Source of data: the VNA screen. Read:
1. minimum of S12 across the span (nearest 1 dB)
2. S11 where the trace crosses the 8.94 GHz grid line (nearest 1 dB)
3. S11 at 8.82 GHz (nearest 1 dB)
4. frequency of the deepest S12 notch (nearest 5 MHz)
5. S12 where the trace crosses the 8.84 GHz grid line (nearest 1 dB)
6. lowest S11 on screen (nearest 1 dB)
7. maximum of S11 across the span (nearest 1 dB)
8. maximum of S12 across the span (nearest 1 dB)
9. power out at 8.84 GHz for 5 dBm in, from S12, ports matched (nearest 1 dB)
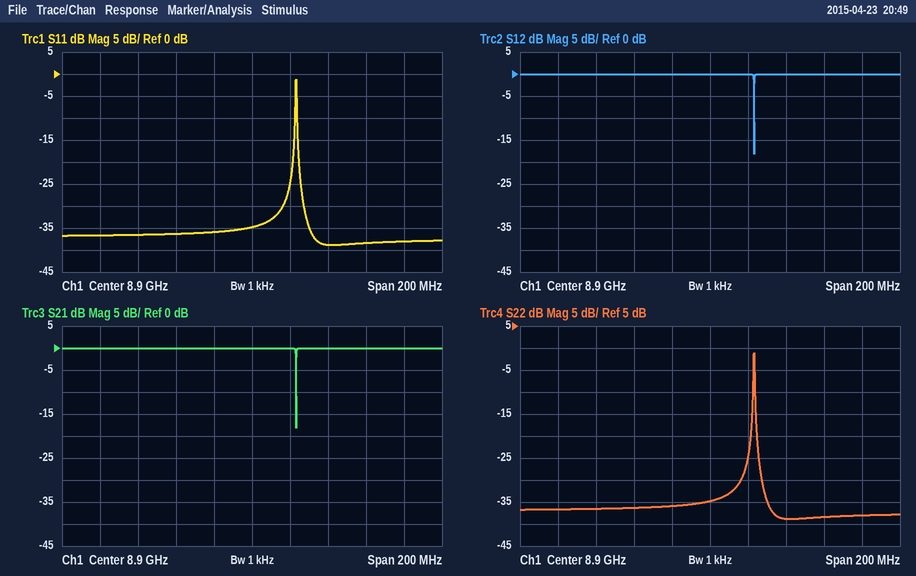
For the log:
-18 dB
-39 dB
-37 dB
8.925 GHz
0 dB
-39 dB
-1 dB
0 dB
5 dBm
